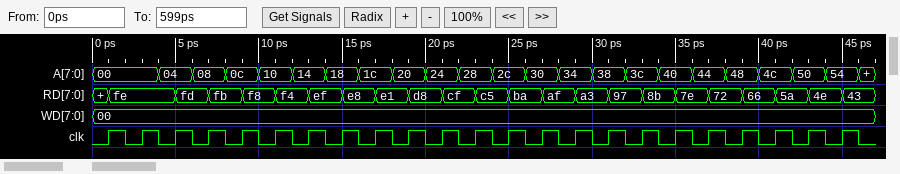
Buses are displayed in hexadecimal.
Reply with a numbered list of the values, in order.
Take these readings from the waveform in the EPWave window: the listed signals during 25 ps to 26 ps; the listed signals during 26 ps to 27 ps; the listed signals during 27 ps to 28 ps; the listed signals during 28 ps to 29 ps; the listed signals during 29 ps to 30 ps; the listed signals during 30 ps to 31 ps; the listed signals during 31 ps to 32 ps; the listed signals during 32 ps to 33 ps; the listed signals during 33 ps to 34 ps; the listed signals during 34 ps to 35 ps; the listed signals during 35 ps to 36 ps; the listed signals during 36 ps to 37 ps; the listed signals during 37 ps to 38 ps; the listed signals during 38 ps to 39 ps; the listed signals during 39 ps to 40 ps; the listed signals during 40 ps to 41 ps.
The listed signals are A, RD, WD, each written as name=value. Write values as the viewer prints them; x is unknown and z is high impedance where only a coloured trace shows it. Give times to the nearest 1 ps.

1. A=2c, RD=ba, WD=00
2. A=30, RD=ba, WD=00
3. A=30, RD=af, WD=00
4. A=34, RD=af, WD=00
5. A=34, RD=a3, WD=00
6. A=38, RD=a3, WD=00
7. A=38, RD=97, WD=00
8. A=3c, RD=97, WD=00
9. A=3c, RD=8b, WD=00
10. A=40, RD=8b, WD=00
11. A=40, RD=7e, WD=00
12. A=44, RD=7e, WD=00
13. A=44, RD=72, WD=00
14. A=48, RD=72, WD=00
15. A=48, RD=66, WD=00
16. A=4c, RD=66, WD=00
